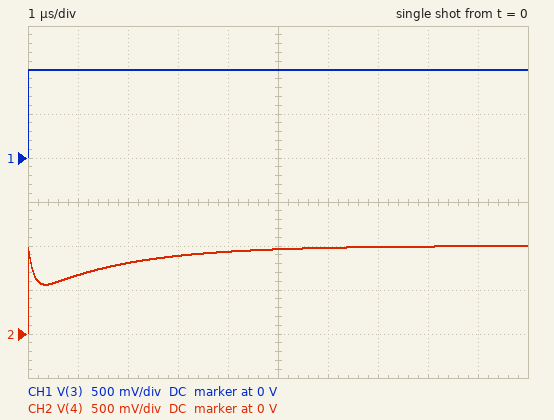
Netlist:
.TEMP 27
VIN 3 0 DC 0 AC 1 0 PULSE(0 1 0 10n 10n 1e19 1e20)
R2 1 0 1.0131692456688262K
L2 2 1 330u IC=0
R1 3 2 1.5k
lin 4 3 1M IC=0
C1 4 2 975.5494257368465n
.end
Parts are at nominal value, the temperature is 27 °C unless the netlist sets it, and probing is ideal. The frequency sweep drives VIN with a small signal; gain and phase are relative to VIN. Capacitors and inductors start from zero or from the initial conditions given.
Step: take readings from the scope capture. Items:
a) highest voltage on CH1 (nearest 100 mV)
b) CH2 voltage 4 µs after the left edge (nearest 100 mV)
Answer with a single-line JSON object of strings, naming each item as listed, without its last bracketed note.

{"highest voltage on CH1": "1.0 V", "CH2 voltage 4 µs after the left edge": "900 mV"}
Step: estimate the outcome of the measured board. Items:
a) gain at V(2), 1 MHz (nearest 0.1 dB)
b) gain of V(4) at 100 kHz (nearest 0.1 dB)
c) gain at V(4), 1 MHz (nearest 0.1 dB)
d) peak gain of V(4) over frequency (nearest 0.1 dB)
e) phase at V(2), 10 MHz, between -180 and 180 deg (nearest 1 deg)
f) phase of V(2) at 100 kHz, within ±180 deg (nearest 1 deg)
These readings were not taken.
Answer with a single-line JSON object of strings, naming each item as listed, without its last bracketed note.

{"gain at V(2), 1 MHz": "-3.4 dB", "gain of V(4) at 100 kHz": "-2.9 dB", "gain at V(4), 1 MHz": "-3.4 dB", "peak gain of V(4) over frequency": "0 dB", "phase at V(2), 10 MHz, between -180 and 180 deg": "4 deg", "phase of V(2) at 100 kHz, within ±180 deg": "-19 deg"}
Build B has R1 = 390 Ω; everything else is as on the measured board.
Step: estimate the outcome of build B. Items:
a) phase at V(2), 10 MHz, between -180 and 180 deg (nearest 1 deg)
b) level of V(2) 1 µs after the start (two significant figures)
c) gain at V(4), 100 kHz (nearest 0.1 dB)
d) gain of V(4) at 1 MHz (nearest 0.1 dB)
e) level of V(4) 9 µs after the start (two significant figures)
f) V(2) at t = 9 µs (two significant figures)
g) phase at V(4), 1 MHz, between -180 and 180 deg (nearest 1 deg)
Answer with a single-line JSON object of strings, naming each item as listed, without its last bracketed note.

{"phase at V(2), 10 MHz, between -180 and 180 deg": "1 deg", "level of V(2) 1 µs after the start": "780 mV", "gain at V(4), 100 kHz": "-2.3 dB", "gain of V(4) at 1 MHz": "-0.8 dB", "level of V(4) 9 µs after the start": "980 mV", "V(2) at t = 9 µs": "970 mV", "phase at V(4), 1 MHz, between -180 and 180 deg": "8 deg"}
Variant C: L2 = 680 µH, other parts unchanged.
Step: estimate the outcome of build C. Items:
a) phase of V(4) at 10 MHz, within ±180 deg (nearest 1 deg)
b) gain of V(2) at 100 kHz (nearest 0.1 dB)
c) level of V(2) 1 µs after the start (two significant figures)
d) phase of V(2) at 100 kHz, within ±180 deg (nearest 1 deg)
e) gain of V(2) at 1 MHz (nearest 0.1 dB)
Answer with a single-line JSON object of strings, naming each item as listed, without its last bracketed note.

{"phase of V(4) at 10 MHz, within ±180 deg": "2 deg", "gain of V(2) at 100 kHz": "-3.1 dB", "level of V(2) 1 µs after the start": "680 mV", "phase of V(2) at 100 kHz, within ±180 deg": "-15 deg", "gain of V(2) at 1 MHz": "-1.5 dB"}
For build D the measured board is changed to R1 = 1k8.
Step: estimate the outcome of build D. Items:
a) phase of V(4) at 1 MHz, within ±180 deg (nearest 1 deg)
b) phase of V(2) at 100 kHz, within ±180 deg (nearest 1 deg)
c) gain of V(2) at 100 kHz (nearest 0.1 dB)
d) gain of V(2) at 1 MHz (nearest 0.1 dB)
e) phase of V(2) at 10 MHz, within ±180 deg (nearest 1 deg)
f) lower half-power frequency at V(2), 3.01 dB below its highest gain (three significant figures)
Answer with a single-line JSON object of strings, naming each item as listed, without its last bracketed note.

{"phase of V(4) at 1 MHz, within ±180 deg": "20 deg", "phase of V(2) at 100 kHz, within ±180 deg": "-21 deg", "gain of V(2) at 100 kHz": "-2.8 dB", "gain of V(2) at 1 MHz": "-4.1 dB", "phase of V(2) at 10 MHz, within ±180 deg": "5 deg", "lower half-power frequency at V(2), 3.01 dB below its highest gain": "216 Hz"}
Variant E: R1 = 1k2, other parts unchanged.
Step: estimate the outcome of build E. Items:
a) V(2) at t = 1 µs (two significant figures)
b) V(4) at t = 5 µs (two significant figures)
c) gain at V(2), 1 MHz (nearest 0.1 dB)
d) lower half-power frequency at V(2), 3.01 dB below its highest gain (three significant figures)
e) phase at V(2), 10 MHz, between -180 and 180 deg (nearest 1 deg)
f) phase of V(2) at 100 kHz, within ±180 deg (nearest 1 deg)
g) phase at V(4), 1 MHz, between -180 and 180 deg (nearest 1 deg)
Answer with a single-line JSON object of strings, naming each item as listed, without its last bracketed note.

{"V(2) at t = 1 µs": "680 mV", "V(4) at t = 5 µs": "960 mV", "gain at V(2), 1 MHz": "-2.7 dB", "lower half-power frequency at V(2), 3.01 dB below its highest gain": "226 Hz", "phase at V(2), 10 MHz, between -180 and 180 deg": "3 deg", "phase of V(2) at 100 kHz, within ±180 deg": "-17 deg", "phase at V(4), 1 MHz, between -180 and 180 deg": "17 deg"}
